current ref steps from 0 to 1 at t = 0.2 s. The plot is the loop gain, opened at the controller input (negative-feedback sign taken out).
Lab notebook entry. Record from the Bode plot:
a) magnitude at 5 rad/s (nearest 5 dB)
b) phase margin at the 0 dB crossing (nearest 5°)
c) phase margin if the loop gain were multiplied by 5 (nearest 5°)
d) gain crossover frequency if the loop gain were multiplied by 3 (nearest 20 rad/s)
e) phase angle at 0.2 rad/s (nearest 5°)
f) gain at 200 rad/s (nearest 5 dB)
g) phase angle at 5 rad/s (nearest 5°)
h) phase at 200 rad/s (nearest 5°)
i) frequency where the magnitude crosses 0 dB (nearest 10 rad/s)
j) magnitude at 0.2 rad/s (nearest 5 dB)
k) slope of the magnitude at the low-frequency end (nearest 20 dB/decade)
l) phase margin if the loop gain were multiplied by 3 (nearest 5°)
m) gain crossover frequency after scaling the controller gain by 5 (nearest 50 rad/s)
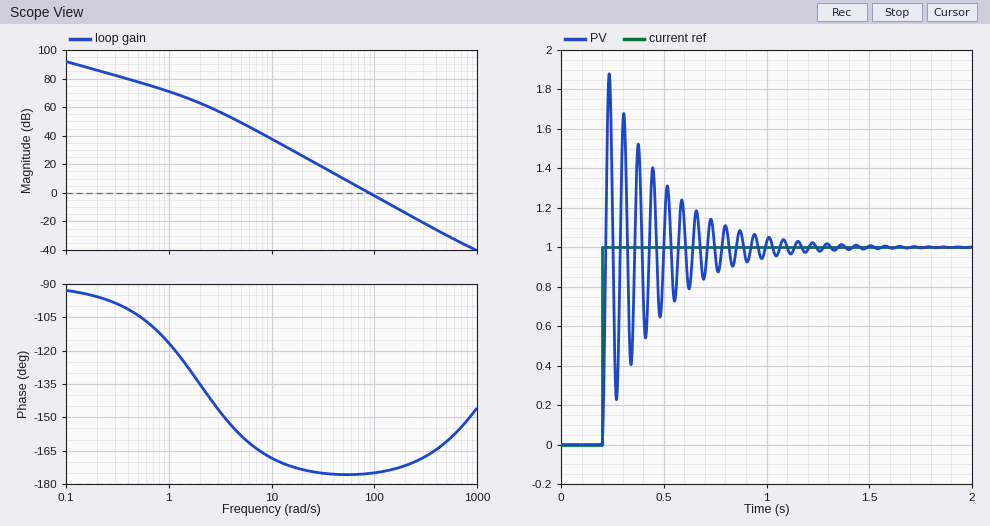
50 dB
5°
10°
160 rad/s
-95°
-15 dB
-160°
-170°
90 rad/s
85 dB
-20 dB/decade
5°
200 rad/s
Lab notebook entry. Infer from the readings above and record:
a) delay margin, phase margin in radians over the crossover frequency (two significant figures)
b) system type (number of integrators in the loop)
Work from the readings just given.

0.00097 s
1
